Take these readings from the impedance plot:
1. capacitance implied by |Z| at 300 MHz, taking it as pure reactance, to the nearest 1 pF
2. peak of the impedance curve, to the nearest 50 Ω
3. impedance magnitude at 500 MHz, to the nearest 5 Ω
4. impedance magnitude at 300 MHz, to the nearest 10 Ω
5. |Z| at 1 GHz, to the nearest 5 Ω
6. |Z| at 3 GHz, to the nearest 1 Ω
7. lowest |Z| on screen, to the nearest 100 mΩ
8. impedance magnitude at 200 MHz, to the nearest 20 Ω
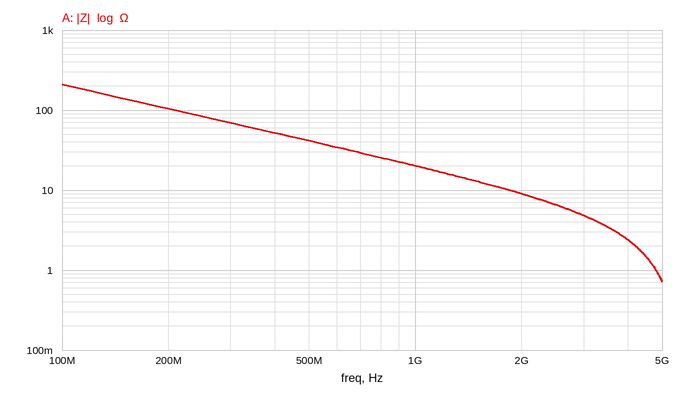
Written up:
8 pF
200 Ω
40 Ω
70 Ω
20 Ω
5 Ω
700 mΩ
100 Ω
